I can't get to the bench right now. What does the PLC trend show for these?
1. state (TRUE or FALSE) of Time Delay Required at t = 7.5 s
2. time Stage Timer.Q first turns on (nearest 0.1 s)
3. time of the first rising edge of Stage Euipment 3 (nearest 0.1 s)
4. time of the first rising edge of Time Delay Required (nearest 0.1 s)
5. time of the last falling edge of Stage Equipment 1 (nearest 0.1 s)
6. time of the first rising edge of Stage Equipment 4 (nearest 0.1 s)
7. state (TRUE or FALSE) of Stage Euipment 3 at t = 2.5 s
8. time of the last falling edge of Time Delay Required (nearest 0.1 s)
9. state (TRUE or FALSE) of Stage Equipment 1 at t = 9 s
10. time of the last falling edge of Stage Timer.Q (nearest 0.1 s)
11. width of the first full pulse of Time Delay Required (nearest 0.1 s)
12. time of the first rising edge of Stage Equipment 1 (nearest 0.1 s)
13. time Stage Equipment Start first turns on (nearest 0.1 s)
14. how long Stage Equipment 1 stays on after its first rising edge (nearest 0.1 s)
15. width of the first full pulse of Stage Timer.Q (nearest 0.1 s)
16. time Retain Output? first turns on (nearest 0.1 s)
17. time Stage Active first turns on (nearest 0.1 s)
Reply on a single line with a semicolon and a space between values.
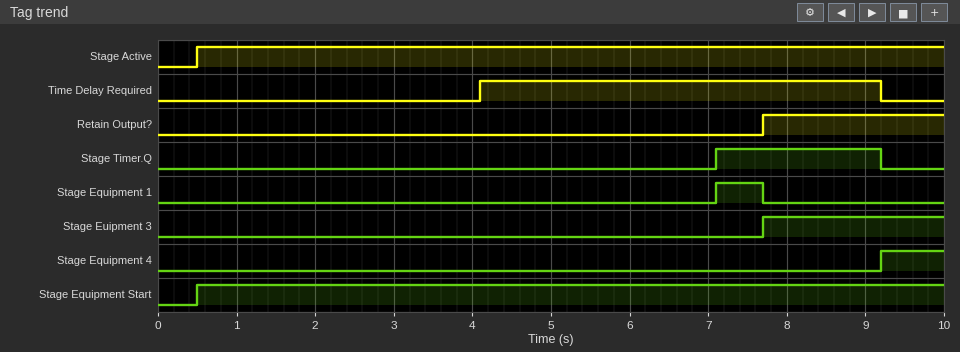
TRUE; 7.1 s; 7.7 s; 4.1 s; 7.7 s; 9.2 s; FALSE; 9.2 s; FALSE; 9.2 s; 5.1 s; 7.1 s; 0.5 s; 0.6 s; 2.1 s; 7.7 s; 0.5 s
